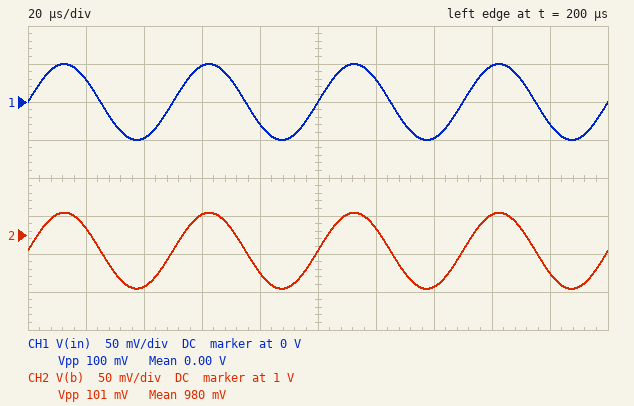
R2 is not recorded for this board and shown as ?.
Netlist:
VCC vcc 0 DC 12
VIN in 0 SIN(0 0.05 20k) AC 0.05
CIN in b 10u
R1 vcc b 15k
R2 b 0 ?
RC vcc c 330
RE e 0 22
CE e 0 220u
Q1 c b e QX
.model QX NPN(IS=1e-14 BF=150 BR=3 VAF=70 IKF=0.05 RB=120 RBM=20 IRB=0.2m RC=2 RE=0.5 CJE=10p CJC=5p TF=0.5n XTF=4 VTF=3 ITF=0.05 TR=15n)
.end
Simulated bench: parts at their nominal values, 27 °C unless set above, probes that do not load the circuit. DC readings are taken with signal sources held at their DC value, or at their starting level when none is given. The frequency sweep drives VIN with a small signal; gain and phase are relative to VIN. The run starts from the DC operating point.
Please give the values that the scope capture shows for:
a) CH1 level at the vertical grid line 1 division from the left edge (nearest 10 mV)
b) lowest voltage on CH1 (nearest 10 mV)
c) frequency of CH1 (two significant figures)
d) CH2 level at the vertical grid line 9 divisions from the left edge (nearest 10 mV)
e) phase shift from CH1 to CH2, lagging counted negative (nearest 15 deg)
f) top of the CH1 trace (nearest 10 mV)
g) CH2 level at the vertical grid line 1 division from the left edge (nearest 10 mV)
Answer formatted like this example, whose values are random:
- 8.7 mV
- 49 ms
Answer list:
- 30 mV
- -50 mV
- 20 kHz
- 950 mV
- 0 deg
- 50 mV
- 1.01 V
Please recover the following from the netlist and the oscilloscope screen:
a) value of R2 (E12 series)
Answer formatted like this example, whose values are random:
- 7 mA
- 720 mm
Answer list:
- 1.5 kΩ
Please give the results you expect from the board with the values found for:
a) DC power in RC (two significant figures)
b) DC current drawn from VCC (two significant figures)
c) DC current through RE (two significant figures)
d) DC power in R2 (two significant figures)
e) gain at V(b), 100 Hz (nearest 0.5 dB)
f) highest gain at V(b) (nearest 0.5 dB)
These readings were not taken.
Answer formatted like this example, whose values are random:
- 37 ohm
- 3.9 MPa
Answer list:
- 41 mW
- 12 mA
- 11 mA
- 640 µW
- -1.0 dB
- 0 dB
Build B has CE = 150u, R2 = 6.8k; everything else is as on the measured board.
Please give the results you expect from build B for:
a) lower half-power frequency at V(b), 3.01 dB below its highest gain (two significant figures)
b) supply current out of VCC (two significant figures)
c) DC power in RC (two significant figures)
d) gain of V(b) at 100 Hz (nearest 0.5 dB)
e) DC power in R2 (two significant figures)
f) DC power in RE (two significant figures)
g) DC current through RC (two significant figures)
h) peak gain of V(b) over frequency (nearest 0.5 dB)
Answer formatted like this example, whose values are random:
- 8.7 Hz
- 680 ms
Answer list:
- 280 Hz
- 34 mA
- 370 mW
- -8.5 dB
- 350 µW
- 25 mW
- 33 mA
- 0 dB
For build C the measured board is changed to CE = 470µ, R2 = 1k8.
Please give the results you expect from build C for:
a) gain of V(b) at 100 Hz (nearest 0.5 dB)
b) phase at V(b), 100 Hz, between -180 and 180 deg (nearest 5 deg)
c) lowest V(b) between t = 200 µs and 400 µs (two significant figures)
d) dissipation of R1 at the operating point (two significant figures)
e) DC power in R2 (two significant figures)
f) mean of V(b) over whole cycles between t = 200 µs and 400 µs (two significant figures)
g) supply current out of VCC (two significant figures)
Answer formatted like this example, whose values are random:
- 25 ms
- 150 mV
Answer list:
- -2.0 dB
- 15 deg
- 1.0 V
- 7.9 mW
- 660 µW
- 1.1 V
- 16 mA
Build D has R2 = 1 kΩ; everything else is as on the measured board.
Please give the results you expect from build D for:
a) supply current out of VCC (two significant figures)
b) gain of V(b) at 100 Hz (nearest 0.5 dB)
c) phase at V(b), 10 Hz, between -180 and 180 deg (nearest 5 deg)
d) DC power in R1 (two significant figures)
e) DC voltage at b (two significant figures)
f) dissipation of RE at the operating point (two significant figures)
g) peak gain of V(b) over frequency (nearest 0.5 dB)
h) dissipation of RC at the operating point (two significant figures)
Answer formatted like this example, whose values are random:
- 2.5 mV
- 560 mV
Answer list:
- 3.3 mA
- -0.5 dB
- 60 deg
- 8.5 mW
- 740 mV
- 140 µW
- 0 dB
- 2.1 mW
